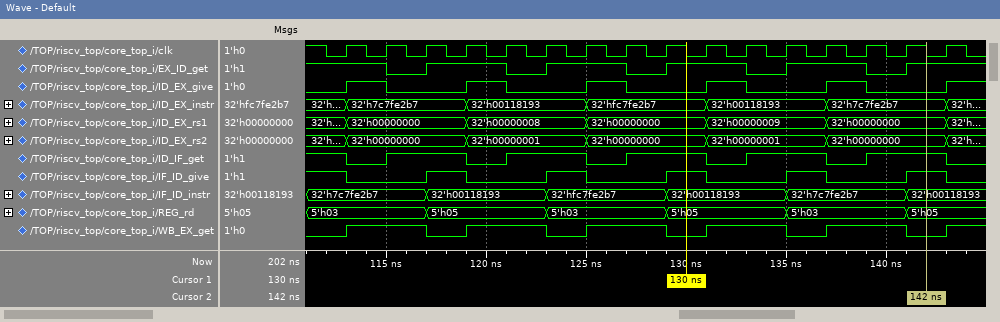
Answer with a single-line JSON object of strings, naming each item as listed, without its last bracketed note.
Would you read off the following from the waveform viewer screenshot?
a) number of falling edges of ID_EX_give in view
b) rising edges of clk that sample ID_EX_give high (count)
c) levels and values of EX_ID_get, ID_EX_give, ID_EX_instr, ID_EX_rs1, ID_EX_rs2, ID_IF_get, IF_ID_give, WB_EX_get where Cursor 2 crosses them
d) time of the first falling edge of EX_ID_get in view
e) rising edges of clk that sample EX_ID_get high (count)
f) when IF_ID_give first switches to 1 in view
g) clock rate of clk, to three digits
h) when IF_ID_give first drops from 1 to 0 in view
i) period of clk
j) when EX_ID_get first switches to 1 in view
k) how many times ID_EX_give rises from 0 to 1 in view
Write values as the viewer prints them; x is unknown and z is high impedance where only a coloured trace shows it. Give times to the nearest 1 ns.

{"number of falling edges of ID_EX_give in view": "5", "rising edges of clk that sample ID_EX_give high": "5", "levels and values of EX_ID_get, ID_EX_give, ID_EX_instr, ID_EX_rs1, ID_EX_rs2, ID_IF_get, IF_ID_give, WB_EX_get where Cursor 2 crosses them": "EX_ID_get=1, ID_EX_give=0, ID_EX_instr=32'h7c7fe2b7, ID_EX_rs1=32'h00000000, ID_EX_rs2=32'h00000000, ID_IF_get=1, IF_ID_give=1, WB_EX_get=0", "time of the first falling edge of EX_ID_get in view": "115 ns", "rising edges of clk that sample EX_ID_get high": "11", "when IF_ID_give first switches to 1 in view": "117 ns", "clock rate of clk, to three digits": "500 MHz", "when IF_ID_give first drops from 1 to 0 in view": "113 ns", "period of clk": "2 ns", "when EX_ID_get first switches to 1 in view": "117 ns", "how many times ID_EX_give rises from 0 to 1 in view": "6"}
